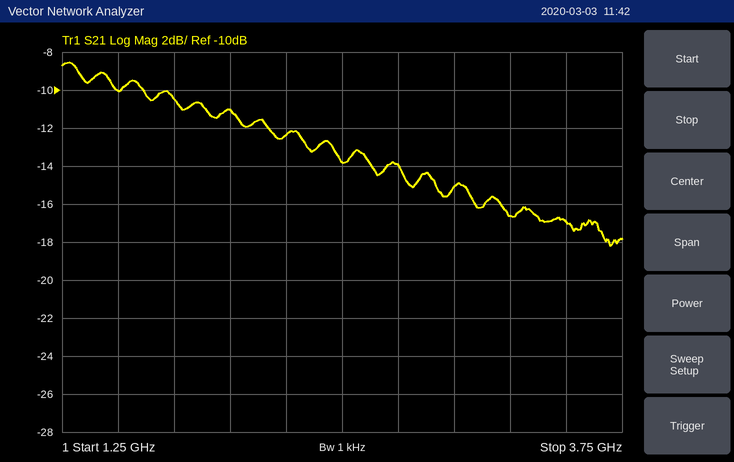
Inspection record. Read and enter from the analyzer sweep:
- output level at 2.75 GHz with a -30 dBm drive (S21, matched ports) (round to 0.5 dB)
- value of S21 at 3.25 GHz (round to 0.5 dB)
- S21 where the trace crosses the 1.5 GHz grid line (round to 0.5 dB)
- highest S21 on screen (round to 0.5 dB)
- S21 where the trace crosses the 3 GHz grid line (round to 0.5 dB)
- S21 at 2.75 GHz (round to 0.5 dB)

-44.0 dBm
-16.5 dB
-10.0 dB
-8.5 dB
-15.0 dB
-14.0 dB
